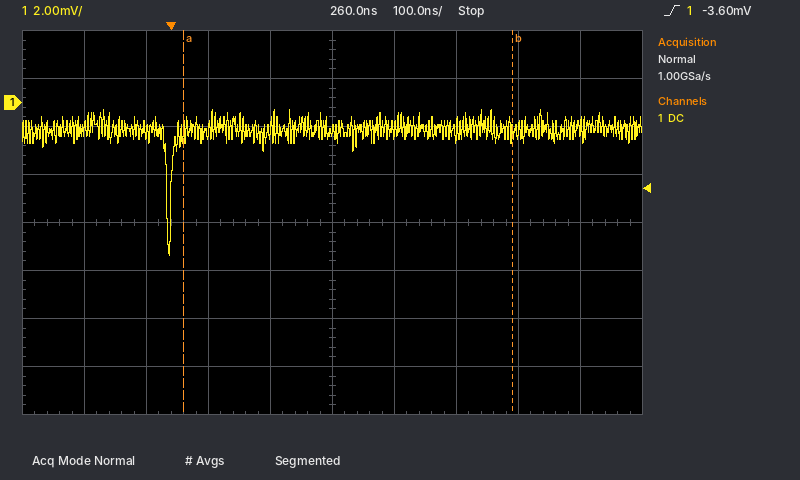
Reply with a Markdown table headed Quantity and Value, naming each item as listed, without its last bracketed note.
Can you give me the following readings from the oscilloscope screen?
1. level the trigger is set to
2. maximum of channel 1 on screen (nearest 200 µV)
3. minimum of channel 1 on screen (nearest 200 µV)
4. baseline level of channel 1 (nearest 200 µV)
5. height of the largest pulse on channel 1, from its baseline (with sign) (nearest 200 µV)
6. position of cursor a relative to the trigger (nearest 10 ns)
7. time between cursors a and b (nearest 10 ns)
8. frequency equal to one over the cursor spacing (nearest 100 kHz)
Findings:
| Quantity | Value |
|---|---|
| level the trigger is set to | -3.60 mV |
| maximum of channel 1 on screen | -200 µV |
| minimum of channel 1 on screen | -6.4 mV |
| baseline level of channel 1 | -1.2 mV |
| height of the largest pulse on channel 1, from its baseline (with sign) | -5.2 mV |
| position of cursor a relative to the trigger | +20 ns |
| time between cursors a and b | 530 ns |
| frequency equal to one over the cursor spacing | 1.9 MHz |
